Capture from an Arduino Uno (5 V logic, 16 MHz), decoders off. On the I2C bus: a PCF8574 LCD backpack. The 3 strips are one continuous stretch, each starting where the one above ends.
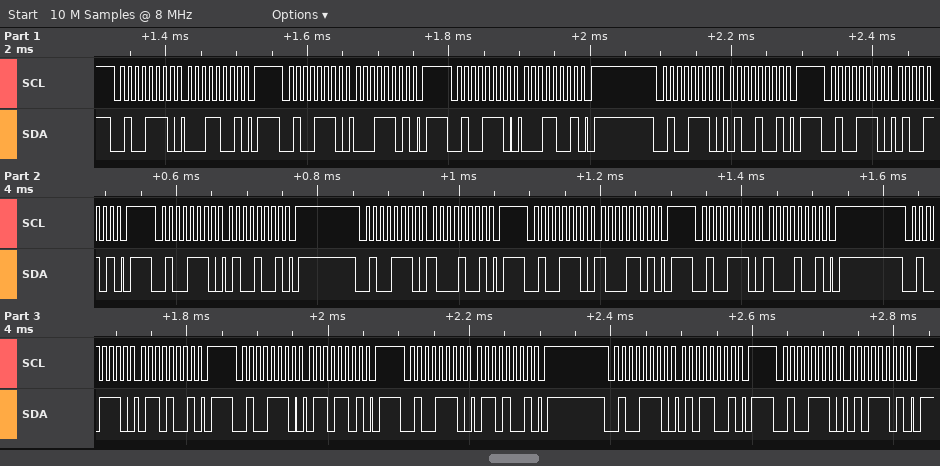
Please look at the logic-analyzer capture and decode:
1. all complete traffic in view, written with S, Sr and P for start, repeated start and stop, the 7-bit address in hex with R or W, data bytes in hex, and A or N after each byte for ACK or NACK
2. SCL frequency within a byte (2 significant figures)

S 27W A 19 A P S 27W A 1D A P S 27W A 19 A P S 27W A 49 A P S 27W A 4D A P S 27W A 49 A P S 27W A 89 A P S 27W A 8D A P S 27W A 89 A P S 27W A 69 A P S 27W A 6D A P S 27W A 69 A P S 27W A 59 A P S 27W A 5D A P
100 kHz
